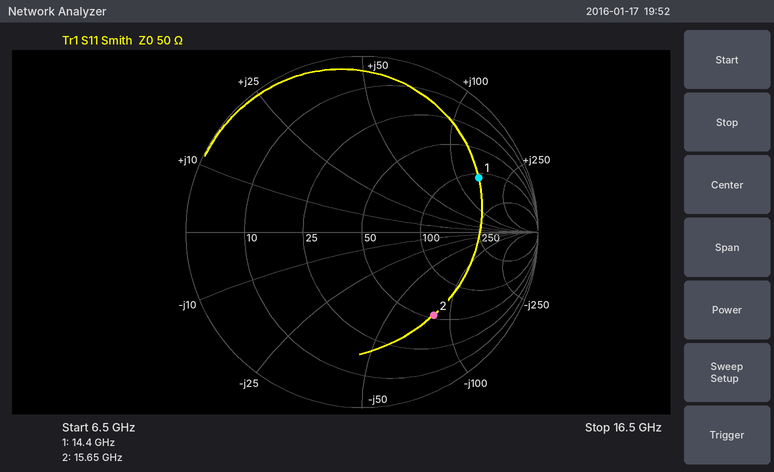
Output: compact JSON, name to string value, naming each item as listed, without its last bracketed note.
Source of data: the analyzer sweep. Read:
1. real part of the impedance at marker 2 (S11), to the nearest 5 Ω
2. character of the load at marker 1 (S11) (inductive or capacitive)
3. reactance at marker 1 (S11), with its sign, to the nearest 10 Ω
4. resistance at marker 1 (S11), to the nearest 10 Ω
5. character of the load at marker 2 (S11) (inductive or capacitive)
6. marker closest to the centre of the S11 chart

{"real part of the impedance at marker 2 (S11), to the nearest 5 Ω": "55 Ω", "character of the load at marker 1 (S11)": "inductive", "reactance at marker 1 (S11), with its sign, to the nearest 10 Ω": "+150 Ω", "resistance at marker 1 (S11), to the nearest 10 Ω": "110 Ω", "character of the load at marker 2 (S11)": "capacitive", "marker closest to the centre of the S11 chart": "marker 2"}
